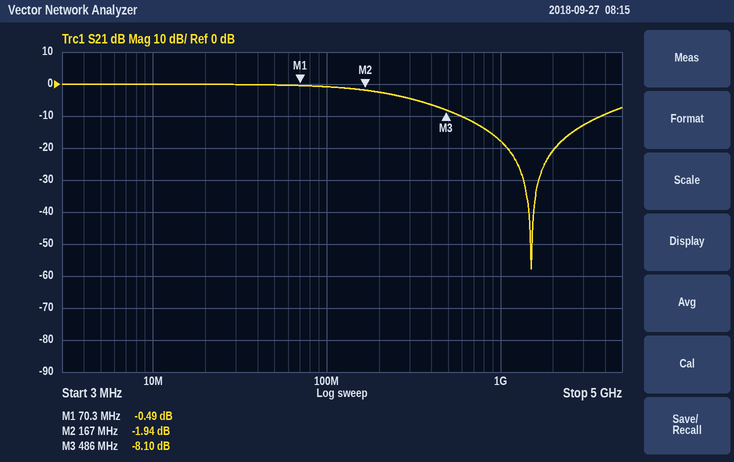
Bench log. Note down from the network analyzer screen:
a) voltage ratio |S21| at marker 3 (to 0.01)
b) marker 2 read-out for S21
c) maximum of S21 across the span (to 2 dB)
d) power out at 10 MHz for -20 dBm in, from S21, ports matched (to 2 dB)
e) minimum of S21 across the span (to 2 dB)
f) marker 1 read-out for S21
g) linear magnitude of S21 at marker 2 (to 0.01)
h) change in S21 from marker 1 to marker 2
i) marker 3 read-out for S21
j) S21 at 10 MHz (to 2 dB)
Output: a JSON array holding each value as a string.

["0.39", "-1.94 dB", "0 dB", "-20 dBm", "-58 dB", "-0.49 dB", "0.80", "-1.45 dB", "-8.10 dB", "0 dB"]
